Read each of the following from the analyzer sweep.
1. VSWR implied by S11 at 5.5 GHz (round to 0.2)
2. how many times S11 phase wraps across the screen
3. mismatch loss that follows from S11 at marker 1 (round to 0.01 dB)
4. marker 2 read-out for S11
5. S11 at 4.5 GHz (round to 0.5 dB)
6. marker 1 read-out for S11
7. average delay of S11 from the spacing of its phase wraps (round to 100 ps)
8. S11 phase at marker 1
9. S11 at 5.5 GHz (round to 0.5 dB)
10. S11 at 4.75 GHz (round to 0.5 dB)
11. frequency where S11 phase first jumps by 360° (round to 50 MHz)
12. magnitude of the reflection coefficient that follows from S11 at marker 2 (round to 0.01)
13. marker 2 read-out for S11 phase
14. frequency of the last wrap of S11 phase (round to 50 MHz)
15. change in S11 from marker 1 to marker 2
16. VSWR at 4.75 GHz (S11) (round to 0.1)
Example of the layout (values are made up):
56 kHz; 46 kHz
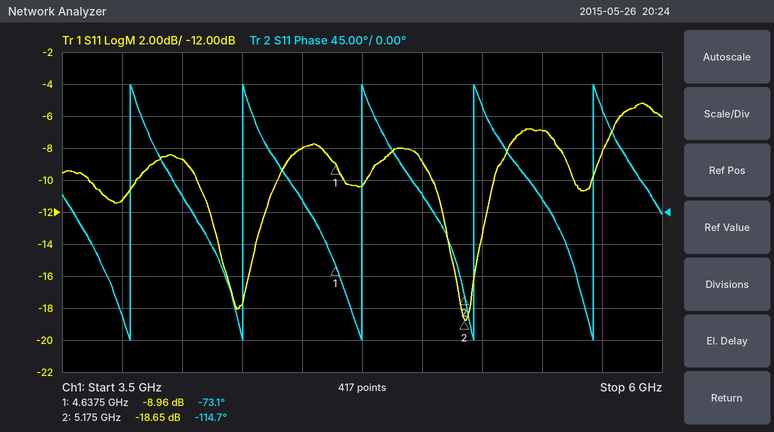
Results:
2.6; 5; 0.59 dB; -18.65 dB; -8.0 dB; -8.96 dB; 2.1 ns; -73.1°; -7.0 dB; -10.5 dB; 3.80 GHz; 0.12; -114.7°; 5.70 GHz; -9.69 dB; 1.9
